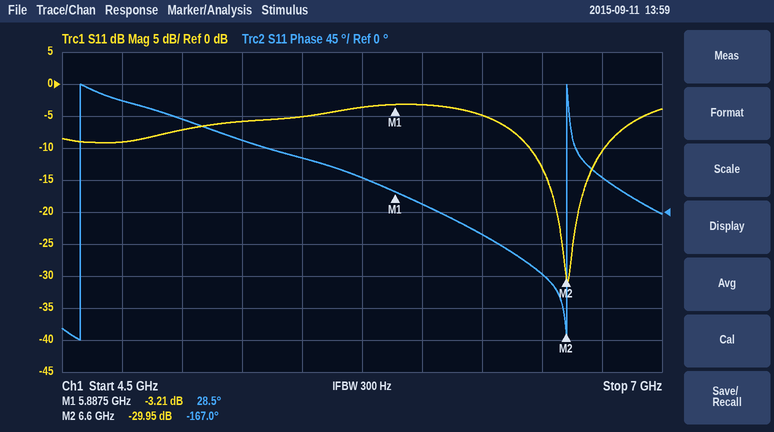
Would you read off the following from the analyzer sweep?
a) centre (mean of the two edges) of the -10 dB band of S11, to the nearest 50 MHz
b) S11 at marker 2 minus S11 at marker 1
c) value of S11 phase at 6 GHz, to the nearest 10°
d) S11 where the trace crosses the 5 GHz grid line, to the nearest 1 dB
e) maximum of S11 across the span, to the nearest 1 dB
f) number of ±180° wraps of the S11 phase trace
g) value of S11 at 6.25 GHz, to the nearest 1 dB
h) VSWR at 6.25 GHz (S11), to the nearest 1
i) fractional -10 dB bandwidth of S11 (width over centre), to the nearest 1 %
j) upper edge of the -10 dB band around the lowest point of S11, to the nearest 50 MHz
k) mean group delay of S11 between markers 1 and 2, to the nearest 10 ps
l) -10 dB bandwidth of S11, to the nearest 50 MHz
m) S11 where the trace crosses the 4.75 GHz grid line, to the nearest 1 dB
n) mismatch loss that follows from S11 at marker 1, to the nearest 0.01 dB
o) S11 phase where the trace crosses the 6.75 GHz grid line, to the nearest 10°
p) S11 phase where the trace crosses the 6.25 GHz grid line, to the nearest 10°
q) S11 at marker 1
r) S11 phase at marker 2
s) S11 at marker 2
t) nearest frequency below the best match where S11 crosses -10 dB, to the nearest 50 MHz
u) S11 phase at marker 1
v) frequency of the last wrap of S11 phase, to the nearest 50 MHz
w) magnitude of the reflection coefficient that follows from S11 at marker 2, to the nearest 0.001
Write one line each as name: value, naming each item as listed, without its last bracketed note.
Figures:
centre (mean of the two edges) of the -10 dB band of S11, to the nearest 50 MHz: 6.60 GHz
S11 at marker 2 minus S11 at marker 1: -26.74 dB
value of S11 phase at 6 GHz, to the nearest 10°: 10°
S11 where the trace crosses the 5 GHz grid line, to the nearest 1 dB: -7 dB
maximum of S11 across the span, to the nearest 1 dB: -3 dB
number of ±180° wraps of the S11 phase trace: 2
value of S11 at 6.25 GHz, to the nearest 1 dB: -5 dB
VSWR at 6.25 GHz (S11), to the nearest 1: 4
fractional -10 dB bandwidth of S11 (width over centre), to the nearest 1 %: 5 %
upper edge of the -10 dB band around the lowest point of S11, to the nearest 50 MHz: 6.75 GHz
mean group delay of S11 between markers 1 and 2, to the nearest 10 ps: 760 ps
-10 dB bandwidth of S11, to the nearest 50 MHz: 300 MHz
S11 where the trace crosses the 4.75 GHz grid line, to the nearest 1 dB: -9 dB
mismatch loss that follows from S11 at marker 1, to the nearest 0.01 dB: 2.82 dB
S11 phase where the trace crosses the 6.75 GHz grid line, to the nearest 10°: 50°
S11 phase where the trace crosses the 6.25 GHz grid line, to the nearest 10°: -30°
S11 at marker 1: -3.21 dB
S11 phase at marker 2: -167.0°
S11 at marker 2: -29.95 dB
nearest frequency below the best match where S11 crosses -10 dB, to the nearest 50 MHz: 6.45 GHz
S11 phase at marker 1: 28.5°
frequency of the last wrap of S11 phase, to the nearest 50 MHz: 6.60 GHz
magnitude of the reflection coefficient that follows from S11 at marker 2, to the nearest 0.001: 0.032
